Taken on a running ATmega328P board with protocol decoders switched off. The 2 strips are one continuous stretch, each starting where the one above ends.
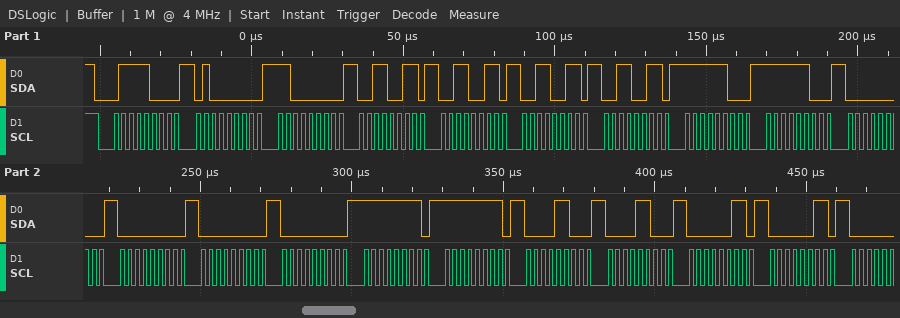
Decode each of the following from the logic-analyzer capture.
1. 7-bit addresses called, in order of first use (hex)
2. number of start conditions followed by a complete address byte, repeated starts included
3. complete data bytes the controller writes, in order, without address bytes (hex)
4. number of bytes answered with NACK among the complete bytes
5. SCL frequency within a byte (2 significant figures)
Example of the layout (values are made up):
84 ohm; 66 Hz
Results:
0x3C; 1; 40 C0 33 33 33 33 FC FC 00 00 00 00 FF FF 0C 0C 03 03; 0; 400 kHz
